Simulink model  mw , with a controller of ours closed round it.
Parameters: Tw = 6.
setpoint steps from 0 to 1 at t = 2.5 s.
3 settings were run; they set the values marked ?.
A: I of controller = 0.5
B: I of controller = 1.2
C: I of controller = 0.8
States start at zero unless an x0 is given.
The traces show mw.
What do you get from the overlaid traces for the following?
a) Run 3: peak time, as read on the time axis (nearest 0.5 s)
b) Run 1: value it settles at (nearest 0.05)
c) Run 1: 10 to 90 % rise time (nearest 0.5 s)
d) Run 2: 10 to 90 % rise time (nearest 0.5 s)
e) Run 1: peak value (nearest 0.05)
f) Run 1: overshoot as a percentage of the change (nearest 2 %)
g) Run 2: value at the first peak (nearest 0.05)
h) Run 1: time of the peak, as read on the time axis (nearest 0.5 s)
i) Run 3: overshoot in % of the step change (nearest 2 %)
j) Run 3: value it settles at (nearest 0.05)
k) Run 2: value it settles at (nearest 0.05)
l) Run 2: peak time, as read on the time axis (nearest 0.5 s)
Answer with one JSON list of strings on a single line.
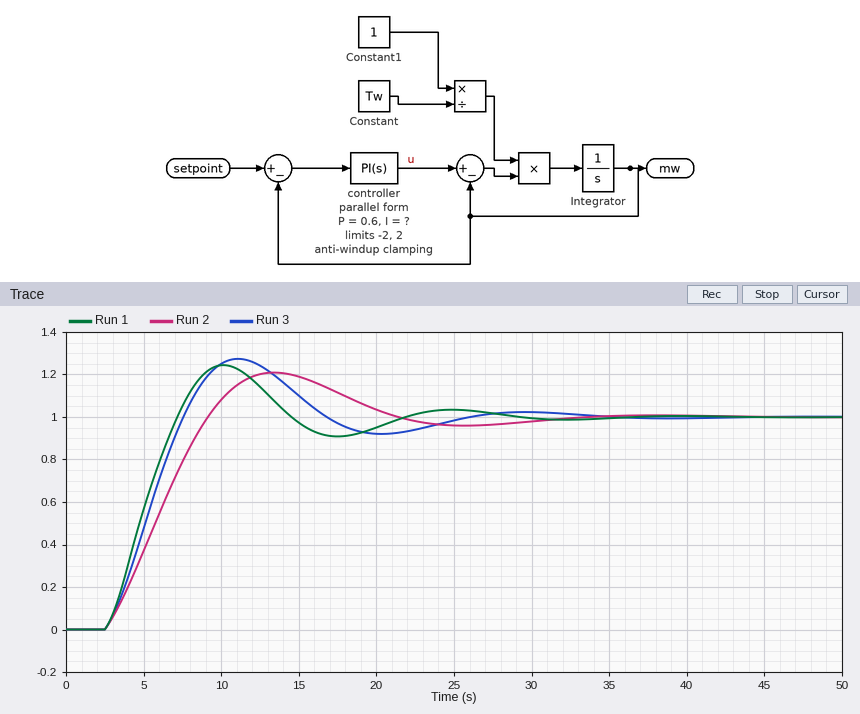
["11.0 s", "1.00", "3.5 s", "5.0 s", "1.25", "24 %", "1.20", "10.0 s", "28 %", "1.00", "1.00", "13.5 s"]
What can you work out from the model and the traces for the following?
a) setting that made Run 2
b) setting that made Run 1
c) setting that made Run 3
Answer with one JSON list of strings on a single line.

["A", "B", "C"]
